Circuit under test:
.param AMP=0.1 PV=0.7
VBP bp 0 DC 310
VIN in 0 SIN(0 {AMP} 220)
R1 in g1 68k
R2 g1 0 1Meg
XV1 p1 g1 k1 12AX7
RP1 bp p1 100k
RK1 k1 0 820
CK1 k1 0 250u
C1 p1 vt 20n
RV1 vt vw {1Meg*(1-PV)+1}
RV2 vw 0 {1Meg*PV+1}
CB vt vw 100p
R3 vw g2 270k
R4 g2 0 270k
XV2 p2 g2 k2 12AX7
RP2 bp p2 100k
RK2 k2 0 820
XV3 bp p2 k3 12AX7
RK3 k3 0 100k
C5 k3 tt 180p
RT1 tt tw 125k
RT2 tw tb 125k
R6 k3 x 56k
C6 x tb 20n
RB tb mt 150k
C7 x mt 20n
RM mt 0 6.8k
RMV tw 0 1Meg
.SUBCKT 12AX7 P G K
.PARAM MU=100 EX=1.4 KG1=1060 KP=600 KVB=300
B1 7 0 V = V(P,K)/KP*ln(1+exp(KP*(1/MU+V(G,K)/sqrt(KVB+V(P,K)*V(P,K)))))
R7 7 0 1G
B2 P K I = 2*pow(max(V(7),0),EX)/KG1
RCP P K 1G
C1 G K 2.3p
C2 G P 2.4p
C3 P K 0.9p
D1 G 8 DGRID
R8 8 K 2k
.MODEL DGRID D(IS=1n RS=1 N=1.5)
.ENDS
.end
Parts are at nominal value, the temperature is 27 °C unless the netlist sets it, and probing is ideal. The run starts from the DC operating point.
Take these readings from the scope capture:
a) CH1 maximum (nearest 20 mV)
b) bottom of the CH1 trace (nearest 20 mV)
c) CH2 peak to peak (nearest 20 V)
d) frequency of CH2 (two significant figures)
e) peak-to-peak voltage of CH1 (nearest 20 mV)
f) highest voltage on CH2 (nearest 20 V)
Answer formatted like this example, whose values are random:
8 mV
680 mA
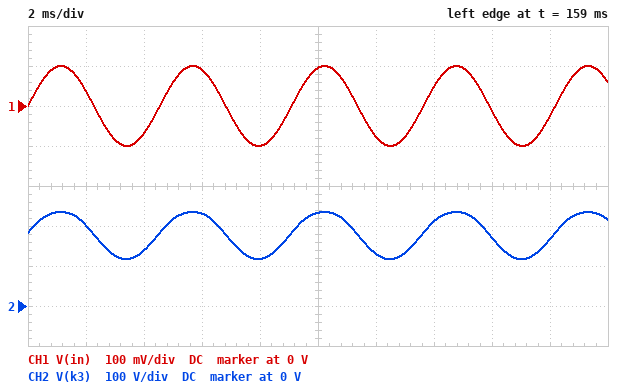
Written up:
100 mV
-100 mV
120 V
220 Hz
200 mV
240 V
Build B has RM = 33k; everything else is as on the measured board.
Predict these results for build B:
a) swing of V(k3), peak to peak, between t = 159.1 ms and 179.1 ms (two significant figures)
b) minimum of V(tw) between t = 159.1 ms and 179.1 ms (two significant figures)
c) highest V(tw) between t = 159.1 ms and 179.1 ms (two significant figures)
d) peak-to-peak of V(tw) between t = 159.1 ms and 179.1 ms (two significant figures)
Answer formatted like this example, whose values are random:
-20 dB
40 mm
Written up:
120 V
-29 V
27 V
56 V
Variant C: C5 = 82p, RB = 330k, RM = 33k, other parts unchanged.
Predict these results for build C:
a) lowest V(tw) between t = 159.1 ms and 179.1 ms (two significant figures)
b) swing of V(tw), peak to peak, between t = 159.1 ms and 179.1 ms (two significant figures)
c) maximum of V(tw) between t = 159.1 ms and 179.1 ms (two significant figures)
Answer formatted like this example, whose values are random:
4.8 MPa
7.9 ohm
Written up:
-28 V
55 V
27 V
